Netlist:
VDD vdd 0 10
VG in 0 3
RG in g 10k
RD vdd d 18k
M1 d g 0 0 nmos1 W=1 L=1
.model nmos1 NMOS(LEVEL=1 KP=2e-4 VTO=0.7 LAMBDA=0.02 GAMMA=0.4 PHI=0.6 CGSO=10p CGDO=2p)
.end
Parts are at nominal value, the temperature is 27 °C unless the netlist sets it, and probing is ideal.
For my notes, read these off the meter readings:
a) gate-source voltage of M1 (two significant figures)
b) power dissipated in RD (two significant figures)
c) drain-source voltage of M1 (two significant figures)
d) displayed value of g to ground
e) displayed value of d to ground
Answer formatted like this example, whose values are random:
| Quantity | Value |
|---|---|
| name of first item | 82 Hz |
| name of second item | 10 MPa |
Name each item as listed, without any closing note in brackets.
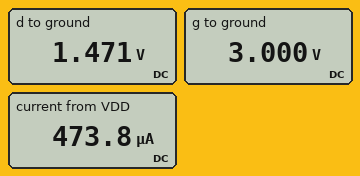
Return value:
| Quantity | Value |
|---|---|
| gate-source voltage of M1 | 3.0 V |
| power dissipated in RD | 4.0 mW |
| drain-source voltage of M1 | 1.5 V |
| displayed value of g to ground | 3.000 V |
| displayed value of d to ground | 1.471 V |
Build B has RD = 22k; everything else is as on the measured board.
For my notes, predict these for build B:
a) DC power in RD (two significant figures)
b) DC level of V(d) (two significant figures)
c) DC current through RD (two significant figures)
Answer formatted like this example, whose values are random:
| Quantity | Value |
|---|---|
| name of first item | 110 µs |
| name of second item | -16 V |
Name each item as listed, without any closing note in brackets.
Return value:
| Quantity | Value |
|---|---|
| DC power in RD | 3.6 mW |
| DC level of V(d) | 1.1 V |
| DC current through RD | 400 µA |
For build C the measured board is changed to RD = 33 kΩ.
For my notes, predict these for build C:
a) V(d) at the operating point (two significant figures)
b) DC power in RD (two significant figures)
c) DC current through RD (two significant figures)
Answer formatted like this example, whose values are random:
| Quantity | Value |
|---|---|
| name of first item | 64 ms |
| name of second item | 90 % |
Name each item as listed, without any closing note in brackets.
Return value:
| Quantity | Value |
|---|---|
| V(d) at the operating point | 710 mV |
| DC power in RD | 2.6 mW |
| DC current through RD | 280 µA |
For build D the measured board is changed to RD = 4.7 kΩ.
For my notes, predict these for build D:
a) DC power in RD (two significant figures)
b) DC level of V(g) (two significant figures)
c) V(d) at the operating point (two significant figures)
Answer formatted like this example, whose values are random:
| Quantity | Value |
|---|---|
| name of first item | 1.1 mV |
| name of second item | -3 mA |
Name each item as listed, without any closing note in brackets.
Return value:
| Quantity | Value |
|---|---|
| DC power in RD | 1.7 mW |
| DC level of V(g) | 3.0 V |
| V(d) at the operating point | 7.2 V |
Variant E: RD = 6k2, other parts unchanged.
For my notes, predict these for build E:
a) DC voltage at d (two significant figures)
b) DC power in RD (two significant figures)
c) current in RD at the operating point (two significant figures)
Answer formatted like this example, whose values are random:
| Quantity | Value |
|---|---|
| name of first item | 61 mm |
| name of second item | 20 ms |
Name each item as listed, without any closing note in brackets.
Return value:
| Quantity | Value |
|---|---|
| DC voltage at d | 6.3 V |
| DC power in RD | 2.2 mW |
| current in RD at the operating point | 600 µA |
